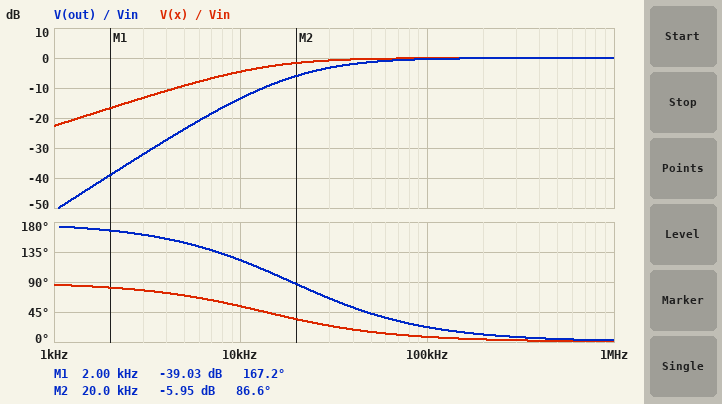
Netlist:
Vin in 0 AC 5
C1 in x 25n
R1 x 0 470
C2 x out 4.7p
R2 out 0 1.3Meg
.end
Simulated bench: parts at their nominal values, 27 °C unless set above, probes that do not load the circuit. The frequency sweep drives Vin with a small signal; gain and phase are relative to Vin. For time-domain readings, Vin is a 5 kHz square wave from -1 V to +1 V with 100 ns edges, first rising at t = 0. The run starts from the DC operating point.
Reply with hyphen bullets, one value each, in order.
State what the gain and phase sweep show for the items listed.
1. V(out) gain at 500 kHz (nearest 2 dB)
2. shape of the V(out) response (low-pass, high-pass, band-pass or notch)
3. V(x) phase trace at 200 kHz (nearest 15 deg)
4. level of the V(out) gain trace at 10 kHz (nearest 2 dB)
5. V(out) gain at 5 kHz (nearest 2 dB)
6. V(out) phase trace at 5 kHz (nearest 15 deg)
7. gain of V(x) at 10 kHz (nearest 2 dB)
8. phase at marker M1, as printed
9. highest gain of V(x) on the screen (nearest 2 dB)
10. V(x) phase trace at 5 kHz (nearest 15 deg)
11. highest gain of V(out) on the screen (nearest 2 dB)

- 0 dB
- high-pass
- 0 deg
- -14 dB
- -24 dB
- 150 deg
- -4 dB
- 167.2 deg
- 0 dB
- 75 deg
- 0 dB
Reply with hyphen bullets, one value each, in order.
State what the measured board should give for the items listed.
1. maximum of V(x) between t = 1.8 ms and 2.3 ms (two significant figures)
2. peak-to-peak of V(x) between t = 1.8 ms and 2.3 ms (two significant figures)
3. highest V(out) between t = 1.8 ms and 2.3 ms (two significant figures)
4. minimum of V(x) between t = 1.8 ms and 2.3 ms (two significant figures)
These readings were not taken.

- 2.0 V
- 4.0 V
- 2.0 V
- -2.0 V
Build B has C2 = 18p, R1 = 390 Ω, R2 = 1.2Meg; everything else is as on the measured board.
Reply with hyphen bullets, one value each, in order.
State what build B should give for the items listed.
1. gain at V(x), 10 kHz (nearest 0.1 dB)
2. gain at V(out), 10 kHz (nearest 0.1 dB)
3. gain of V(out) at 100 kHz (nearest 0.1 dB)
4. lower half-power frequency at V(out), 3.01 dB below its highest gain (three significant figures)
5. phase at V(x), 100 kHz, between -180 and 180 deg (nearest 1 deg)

- -5.6 dB
- -7.5 dB
- -0.1 dB
- 19.0 kHz
- 9 deg
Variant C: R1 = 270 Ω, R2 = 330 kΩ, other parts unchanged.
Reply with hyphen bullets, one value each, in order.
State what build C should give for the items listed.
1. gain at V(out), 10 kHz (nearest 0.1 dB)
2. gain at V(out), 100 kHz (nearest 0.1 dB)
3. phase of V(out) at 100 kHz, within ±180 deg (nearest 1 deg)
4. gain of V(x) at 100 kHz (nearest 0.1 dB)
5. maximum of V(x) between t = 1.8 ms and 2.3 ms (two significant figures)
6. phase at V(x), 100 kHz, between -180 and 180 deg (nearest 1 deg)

- -28.4 dB
- -3.4 dB
- 59 deg
- -0.2 dB
- 2.0 V
- 13 deg
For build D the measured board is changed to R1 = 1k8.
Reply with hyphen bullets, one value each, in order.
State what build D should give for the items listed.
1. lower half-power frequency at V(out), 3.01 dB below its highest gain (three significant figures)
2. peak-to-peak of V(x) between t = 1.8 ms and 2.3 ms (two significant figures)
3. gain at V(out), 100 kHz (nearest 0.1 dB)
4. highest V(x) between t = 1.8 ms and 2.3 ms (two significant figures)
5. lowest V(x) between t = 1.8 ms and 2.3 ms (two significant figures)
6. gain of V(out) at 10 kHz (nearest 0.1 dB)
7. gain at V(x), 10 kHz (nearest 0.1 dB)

- 26.5 kHz
- 3.6 V
- -0.3 dB
- 1.8 V
- -1.8 V
- -9.4 dB
- -0.5 dB
